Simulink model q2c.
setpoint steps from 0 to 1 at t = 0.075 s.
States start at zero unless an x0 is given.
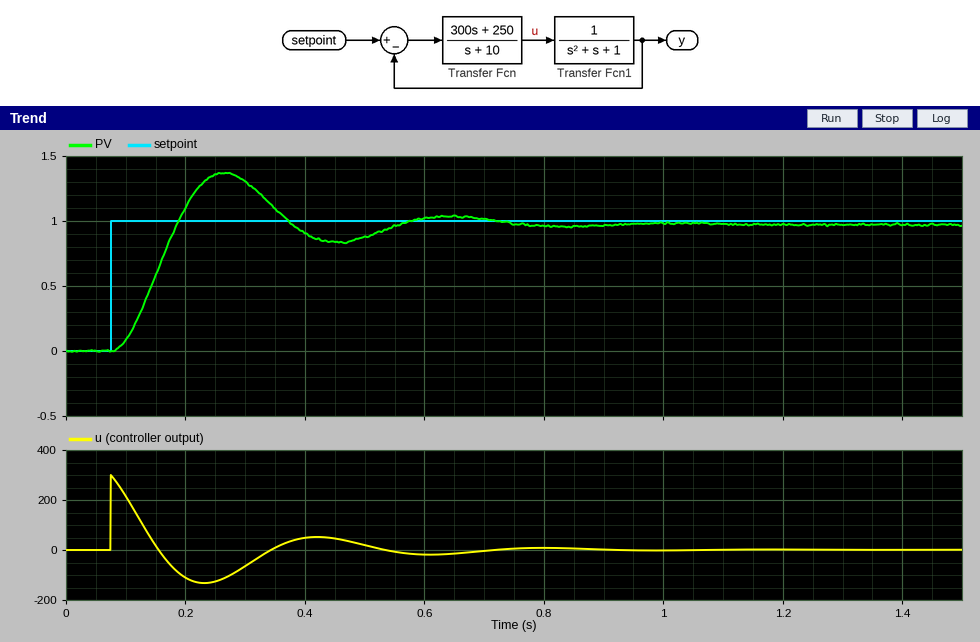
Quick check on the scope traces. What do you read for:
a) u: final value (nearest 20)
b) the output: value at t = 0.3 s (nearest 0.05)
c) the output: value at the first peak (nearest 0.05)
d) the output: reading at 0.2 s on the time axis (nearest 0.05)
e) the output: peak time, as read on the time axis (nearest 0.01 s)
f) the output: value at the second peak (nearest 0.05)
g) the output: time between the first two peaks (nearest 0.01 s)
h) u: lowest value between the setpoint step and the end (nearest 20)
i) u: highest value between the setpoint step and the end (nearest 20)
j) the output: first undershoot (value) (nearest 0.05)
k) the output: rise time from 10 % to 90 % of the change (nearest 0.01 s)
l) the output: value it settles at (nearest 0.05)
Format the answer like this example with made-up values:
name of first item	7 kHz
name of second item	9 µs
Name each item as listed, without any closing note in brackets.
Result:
u: final value	0
the output: value at t = 0.3 s	1.30
the output: value at the first peak	1.35
the output: reading at 0.2 s on the time axis	1.10
the output: peak time, as read on the time axis	0.26 s
the output: value at the second peak	1.05
the output: time between the first two peaks	0.38 s
u: lowest value between the setpoint step and the end	-140
u: highest value between the setpoint step and the end	300
the output: first undershoot (value)	0.85
the output: rise time from 10 % to 90 % of the change	0.07 s
the output: value it settles at	0.95
